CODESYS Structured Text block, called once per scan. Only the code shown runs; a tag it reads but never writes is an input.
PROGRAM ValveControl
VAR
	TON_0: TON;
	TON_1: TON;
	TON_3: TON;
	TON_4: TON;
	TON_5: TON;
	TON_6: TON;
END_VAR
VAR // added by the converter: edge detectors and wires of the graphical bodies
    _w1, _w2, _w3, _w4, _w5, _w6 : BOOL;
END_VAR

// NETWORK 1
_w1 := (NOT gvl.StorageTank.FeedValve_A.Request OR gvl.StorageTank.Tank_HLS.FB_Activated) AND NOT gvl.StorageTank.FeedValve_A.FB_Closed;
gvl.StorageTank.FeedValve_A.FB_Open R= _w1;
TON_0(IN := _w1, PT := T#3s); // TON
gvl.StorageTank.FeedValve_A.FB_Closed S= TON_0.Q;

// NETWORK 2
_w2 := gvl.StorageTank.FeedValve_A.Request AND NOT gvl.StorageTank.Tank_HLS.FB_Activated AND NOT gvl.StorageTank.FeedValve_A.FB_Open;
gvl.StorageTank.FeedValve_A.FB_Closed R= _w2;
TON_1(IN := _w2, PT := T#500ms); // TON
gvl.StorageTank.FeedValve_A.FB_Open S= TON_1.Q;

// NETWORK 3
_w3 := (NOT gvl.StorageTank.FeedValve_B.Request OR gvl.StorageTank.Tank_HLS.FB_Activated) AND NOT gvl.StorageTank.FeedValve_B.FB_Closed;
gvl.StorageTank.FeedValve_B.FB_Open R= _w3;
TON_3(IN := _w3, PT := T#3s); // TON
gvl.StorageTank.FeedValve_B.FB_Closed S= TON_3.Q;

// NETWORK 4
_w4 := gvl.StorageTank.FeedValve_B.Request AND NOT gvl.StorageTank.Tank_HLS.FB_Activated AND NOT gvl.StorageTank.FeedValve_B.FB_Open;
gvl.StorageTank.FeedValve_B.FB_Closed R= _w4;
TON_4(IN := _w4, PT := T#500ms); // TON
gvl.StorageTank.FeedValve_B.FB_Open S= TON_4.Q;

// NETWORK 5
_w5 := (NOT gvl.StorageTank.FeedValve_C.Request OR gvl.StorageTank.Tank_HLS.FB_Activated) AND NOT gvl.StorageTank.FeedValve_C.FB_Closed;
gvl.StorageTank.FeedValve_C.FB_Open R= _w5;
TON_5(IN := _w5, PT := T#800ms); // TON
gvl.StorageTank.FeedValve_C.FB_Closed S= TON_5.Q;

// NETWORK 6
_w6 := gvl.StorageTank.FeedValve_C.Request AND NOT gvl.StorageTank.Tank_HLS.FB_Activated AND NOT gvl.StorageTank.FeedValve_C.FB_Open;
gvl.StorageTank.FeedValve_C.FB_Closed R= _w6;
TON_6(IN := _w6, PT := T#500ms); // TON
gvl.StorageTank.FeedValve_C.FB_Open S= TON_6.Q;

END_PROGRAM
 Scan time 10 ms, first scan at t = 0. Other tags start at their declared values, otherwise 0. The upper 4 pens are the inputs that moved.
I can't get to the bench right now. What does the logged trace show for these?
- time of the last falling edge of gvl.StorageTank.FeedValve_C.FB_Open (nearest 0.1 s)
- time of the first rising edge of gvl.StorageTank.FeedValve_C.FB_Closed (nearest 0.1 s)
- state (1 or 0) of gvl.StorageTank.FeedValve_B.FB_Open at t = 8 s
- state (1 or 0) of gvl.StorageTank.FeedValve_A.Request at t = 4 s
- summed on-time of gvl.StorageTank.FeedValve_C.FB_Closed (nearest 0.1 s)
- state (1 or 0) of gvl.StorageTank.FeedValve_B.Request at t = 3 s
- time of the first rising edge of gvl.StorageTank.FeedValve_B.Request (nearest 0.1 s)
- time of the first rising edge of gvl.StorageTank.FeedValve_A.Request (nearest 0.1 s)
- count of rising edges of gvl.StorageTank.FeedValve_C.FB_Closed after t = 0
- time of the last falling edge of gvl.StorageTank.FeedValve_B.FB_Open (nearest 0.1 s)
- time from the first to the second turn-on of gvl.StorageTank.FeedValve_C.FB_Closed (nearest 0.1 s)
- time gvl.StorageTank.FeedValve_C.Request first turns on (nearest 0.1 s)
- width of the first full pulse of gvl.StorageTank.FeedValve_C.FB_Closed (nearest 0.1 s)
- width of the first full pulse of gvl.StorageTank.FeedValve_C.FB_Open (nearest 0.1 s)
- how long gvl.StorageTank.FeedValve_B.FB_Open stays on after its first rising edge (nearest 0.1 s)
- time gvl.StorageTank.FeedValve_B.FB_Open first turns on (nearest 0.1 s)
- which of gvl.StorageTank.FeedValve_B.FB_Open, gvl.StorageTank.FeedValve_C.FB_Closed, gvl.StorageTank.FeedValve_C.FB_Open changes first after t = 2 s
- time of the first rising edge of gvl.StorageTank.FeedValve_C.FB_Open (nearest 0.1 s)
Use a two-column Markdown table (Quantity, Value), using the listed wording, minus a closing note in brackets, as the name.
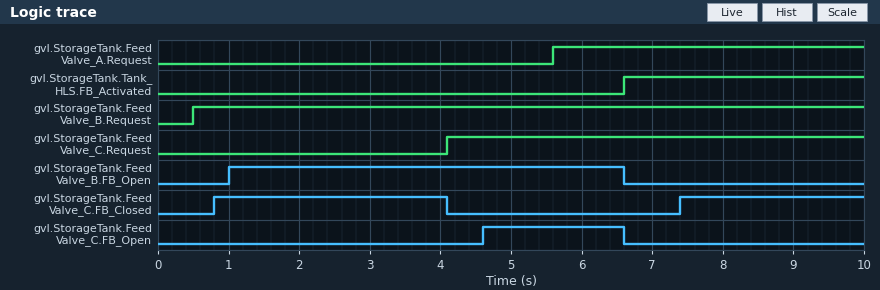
| Quantity | Value |
|---|---|
| time of the last falling edge of gvl.StorageTank.FeedValve_C.FB_Open | 6.6 s |
| time of the first rising edge of gvl.StorageTank.FeedValve_C.FB_Closed | 0.8 s |
| state (1 or 0) of gvl.StorageTank.FeedValve_B.FB_Open at t = 8 s | 0 |
| state (1 or 0) of gvl.StorageTank.FeedValve_A.Request at t = 4 s | 0 |
| summed on-time of gvl.StorageTank.FeedValve_C.FB_Closed | 5.9 s |
| state (1 or 0) of gvl.StorageTank.FeedValve_B.Request at t = 3 s | 1 |
| time of the first rising edge of gvl.StorageTank.FeedValve_B.Request | 0.5 s |
| time of the first rising edge of gvl.StorageTank.FeedValve_A.Request | 5.6 s |
| count of rising edges of gvl.StorageTank.FeedValve_C.FB_Closed after t = 0 | 2 |
| time of the last falling edge of gvl.StorageTank.FeedValve_B.FB_Open | 6.6 s |
| time from the first to the second turn-on of gvl.StorageTank.FeedValve_C.FB_Closed | 6.6 s |
| time gvl.StorageTank.FeedValve_C.Request first turns on | 4.1 s |
| width of the first full pulse of gvl.StorageTank.FeedValve_C.FB_Closed | 3.3 s |
| width of the first full pulse of gvl.StorageTank.FeedValve_C.FB_Open | 2.0 s |
| how long gvl.StorageTank.FeedValve_B.FB_Open stays on after its first rising edge | 5.6 s |
| time gvl.StorageTank.FeedValve_B.FB_Open first turns on | 1.0 s |
| which of gvl.StorageTank.FeedValve_B.FB_Open, gvl.StorageTank.FeedValve_C.FB_Closed, gvl.StorageTank.FeedValve_C.FB_Open changes first after t = 2 s | gvl.StorageTank.FeedValve_C.FB_Closed |
| time of the first rising edge of gvl.StorageTank.FeedValve_C.FB_Open | 4.6 s |
